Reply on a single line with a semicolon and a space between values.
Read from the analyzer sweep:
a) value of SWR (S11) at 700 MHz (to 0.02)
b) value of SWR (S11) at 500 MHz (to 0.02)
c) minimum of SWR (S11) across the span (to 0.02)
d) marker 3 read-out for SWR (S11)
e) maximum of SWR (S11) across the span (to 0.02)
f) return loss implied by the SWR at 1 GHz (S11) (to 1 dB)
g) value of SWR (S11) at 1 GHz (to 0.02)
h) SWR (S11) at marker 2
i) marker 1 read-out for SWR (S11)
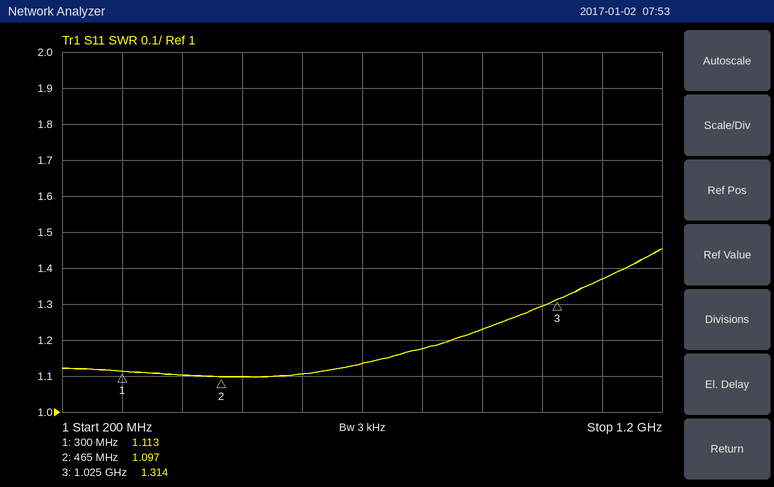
1.14; 1.10; 1.10; 1.314; 1.46; 18 dB; 1.30; 1.097; 1.113
